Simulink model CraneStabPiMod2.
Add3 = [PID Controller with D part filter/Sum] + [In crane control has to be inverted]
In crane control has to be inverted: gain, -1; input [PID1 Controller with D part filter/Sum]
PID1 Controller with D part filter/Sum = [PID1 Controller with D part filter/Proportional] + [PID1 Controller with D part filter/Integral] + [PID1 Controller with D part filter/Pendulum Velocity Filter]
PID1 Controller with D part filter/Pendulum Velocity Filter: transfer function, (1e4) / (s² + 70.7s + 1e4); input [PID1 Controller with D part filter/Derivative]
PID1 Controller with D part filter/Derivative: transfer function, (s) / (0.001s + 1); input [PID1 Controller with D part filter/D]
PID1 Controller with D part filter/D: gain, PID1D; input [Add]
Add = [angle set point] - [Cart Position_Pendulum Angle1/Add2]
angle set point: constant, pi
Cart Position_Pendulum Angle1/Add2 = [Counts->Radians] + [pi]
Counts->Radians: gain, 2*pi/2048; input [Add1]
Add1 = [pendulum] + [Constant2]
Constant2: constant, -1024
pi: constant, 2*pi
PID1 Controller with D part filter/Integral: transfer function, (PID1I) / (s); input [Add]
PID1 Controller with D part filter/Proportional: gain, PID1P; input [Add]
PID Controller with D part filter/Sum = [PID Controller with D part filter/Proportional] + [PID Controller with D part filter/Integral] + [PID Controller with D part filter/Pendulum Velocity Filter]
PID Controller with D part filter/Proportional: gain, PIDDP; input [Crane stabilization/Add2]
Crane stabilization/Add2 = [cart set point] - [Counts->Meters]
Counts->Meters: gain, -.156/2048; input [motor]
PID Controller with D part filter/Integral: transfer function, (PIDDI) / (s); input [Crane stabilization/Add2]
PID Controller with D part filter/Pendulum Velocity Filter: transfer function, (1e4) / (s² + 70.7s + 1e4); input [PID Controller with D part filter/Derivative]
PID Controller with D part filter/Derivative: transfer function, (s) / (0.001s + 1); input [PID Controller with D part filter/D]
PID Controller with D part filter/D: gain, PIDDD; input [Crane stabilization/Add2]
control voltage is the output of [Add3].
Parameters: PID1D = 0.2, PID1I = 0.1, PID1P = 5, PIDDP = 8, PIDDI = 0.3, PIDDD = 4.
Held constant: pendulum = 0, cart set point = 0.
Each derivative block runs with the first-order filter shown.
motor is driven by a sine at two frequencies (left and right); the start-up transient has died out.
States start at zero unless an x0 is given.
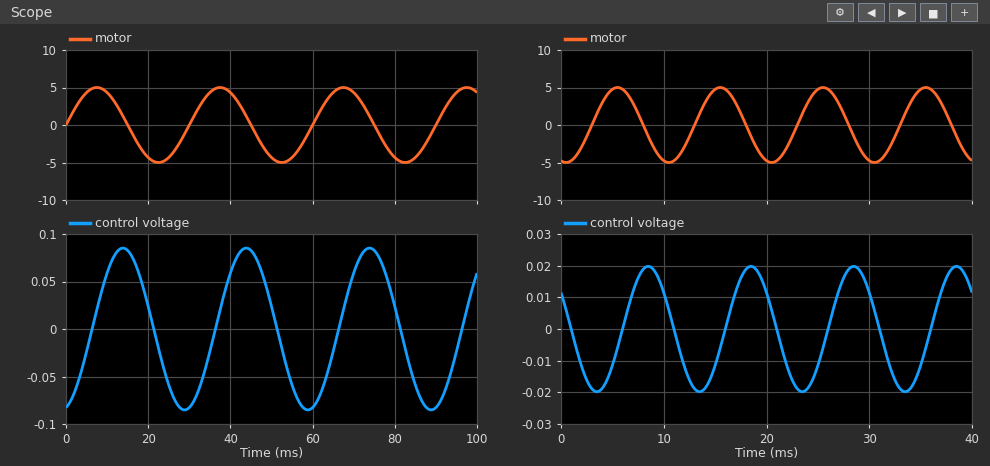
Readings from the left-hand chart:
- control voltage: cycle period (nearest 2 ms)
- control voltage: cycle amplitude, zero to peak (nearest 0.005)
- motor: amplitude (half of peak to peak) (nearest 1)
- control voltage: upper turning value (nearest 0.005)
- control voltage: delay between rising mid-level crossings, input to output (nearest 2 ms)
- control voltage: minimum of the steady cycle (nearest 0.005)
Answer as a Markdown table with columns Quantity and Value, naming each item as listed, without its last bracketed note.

| Quantity | Value |
|---|---|
| control voltage: cycle period | 30 ms |
| control voltage: cycle amplitude, zero to peak | 0.085 |
| motor: amplitude (half of peak to peak) | 5 |
| control voltage: upper turning value | 0.085 |
| control voltage: delay between rising mid-level crossings, input to output | 6 ms |
| control voltage: minimum of the steady cycle | -0.085 |
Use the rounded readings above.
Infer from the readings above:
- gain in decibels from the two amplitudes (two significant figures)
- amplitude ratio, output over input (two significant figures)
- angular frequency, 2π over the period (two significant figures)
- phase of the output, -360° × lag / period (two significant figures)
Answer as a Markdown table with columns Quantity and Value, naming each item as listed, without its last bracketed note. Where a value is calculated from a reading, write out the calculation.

| Quantity | Value |
|---|---|
| gain in decibels from the two amplitudes | 20 log10(0.085 / 5) = -35 dB |
| amplitude ratio, output over input | 0.085 / 5 = 0.017 |
| angular frequency, 2π over the period | 2π / 30 = 0.21 rad/ms |
| phase of the output, -360° × lag / period | -360 × 6 / 30 = -72° |
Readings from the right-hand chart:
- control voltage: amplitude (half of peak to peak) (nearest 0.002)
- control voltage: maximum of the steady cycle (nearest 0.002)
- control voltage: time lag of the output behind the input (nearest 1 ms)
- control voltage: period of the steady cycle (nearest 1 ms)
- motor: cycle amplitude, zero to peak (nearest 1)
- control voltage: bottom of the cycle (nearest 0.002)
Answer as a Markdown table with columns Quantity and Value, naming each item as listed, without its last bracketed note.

| Quantity | Value |
|---|---|
| control voltage: amplitude (half of peak to peak) | 0.020 |
| control voltage: maximum of the steady cycle | 0.020 |
| control voltage: time lag of the output behind the input | 3 ms |
| control voltage: period of the steady cycle | 10 ms |
| motor: cycle amplitude, zero to peak | 5 |
| control voltage: bottom of the cycle | -0.020 |
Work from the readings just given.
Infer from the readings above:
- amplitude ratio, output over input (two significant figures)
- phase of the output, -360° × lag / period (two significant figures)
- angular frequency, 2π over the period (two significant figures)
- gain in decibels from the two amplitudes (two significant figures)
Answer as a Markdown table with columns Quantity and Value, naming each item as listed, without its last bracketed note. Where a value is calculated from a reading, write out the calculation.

| Quantity | Value |
|---|---|
| amplitude ratio, output over input | 0.02 / 5 = 0.0040 |
| phase of the output, -360° × lag / period | -360 × 3 / 10 = -110° |
| angular frequency, 2π over the period | 2π / 10 = 0.63 rad/ms |
| gain in decibels from the two amplitudes | 20 log10(0.02 / 5) = -48 dB |
